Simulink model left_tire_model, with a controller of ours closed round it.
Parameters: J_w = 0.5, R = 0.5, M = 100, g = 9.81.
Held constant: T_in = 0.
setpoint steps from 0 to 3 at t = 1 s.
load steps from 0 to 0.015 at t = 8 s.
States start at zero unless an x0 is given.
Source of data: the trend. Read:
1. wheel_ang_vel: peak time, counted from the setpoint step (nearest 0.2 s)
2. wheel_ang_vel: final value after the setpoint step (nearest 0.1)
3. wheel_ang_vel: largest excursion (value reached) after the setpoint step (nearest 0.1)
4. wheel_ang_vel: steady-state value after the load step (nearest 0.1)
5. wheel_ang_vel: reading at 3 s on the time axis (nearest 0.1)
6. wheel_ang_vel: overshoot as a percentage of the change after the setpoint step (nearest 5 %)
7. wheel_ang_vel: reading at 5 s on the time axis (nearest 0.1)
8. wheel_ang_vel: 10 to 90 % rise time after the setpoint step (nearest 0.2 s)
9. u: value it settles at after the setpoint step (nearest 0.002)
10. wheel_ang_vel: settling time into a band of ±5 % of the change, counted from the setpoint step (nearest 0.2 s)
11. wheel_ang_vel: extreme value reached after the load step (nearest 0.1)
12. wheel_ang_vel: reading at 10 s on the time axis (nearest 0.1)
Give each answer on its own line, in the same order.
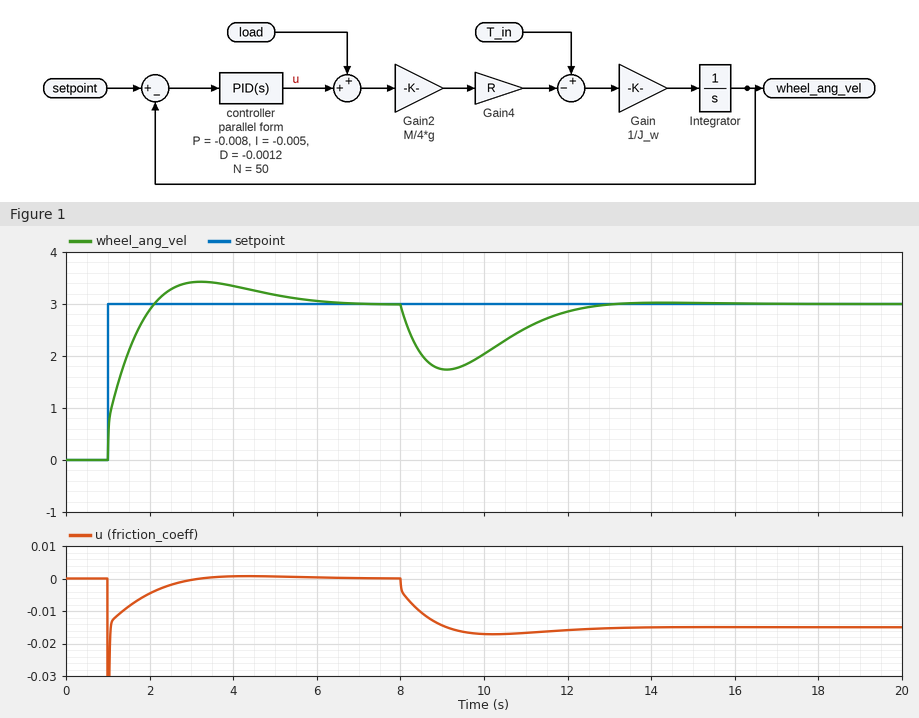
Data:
2.2 s
3.0
3.4
3.0
3.4
15 %
3.2
0.8 s
0.000
4.2 s
1.7
2.0
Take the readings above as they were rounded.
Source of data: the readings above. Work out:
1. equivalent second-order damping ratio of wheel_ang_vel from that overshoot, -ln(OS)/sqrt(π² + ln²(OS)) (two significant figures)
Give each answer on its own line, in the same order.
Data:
0.52
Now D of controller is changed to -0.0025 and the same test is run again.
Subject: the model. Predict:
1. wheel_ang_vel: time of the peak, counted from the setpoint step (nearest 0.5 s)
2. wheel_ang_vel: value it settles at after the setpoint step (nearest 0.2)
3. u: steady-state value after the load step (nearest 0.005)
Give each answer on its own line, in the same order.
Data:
2.5 s
3.0
-0.015
